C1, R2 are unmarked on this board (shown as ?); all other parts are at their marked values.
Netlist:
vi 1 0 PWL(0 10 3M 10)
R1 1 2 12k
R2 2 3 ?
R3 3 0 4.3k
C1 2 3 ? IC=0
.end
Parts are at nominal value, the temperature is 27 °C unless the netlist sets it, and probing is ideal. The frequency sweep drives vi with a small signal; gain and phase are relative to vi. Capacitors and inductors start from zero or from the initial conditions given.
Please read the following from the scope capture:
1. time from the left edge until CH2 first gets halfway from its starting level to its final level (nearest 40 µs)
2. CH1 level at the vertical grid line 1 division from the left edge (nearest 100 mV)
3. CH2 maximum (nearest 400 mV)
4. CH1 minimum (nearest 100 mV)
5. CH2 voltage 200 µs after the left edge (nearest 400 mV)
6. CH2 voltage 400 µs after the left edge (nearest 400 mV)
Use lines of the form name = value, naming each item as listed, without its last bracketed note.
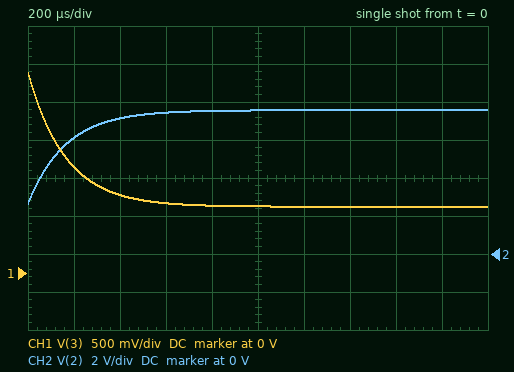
time from the left edge until CH2 first gets halfway from its starting level to its final level = 120 µs
CH1 level at the vertical grid line 1 division from the left edge = 1.4 V
CH2 maximum = 7.6 V
CH1 minimum = 900 mV
CH2 voltage 200 µs after the left edge = 6.0 V
CH2 voltage 400 µs after the left edge = 7.2 V
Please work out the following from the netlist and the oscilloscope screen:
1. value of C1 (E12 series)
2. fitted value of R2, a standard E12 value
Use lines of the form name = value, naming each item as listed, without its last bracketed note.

value of C1 = 15 nF
fitted value of R2, a standard E12 value = 33 kΩ
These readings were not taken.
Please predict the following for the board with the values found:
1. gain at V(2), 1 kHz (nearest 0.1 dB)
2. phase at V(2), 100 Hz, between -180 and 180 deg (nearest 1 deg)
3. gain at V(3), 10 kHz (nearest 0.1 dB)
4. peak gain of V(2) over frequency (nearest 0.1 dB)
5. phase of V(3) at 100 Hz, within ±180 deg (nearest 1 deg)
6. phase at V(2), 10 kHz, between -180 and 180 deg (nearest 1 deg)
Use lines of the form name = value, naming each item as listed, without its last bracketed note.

gain at V(2), 1 kHz = -5.0 dB
phase at V(2), 100 Hz, between -180 and 180 deg = -4 deg
gain at V(3), 10 kHz = -11.6 dB
peak gain of V(2) over frequency = -2.4 dB
phase of V(3) at 100 Hz, within ±180 deg = 11 deg
phase at V(2), 10 kHz, between -180 and 180 deg = -10 deg
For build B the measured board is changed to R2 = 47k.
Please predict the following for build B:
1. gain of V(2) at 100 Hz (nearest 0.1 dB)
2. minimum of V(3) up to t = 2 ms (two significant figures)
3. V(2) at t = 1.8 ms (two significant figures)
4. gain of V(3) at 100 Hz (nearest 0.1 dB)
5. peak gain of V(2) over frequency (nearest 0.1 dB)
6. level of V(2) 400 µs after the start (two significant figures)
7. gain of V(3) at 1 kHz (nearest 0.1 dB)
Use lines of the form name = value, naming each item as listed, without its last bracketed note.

gain of V(2) at 100 Hz = -1.9 dB
minimum of V(3) up to t = 2 ms = 680 mV
V(2) at t = 1.8 ms = 8.1 V
gain of V(3) at 100 Hz = -22.6 dB
peak gain of V(2) over frequency = -1.8 dB
level of V(2) 400 µs after the start = 7.5 V
gain of V(3) at 1 kHz = -13.8 dB
